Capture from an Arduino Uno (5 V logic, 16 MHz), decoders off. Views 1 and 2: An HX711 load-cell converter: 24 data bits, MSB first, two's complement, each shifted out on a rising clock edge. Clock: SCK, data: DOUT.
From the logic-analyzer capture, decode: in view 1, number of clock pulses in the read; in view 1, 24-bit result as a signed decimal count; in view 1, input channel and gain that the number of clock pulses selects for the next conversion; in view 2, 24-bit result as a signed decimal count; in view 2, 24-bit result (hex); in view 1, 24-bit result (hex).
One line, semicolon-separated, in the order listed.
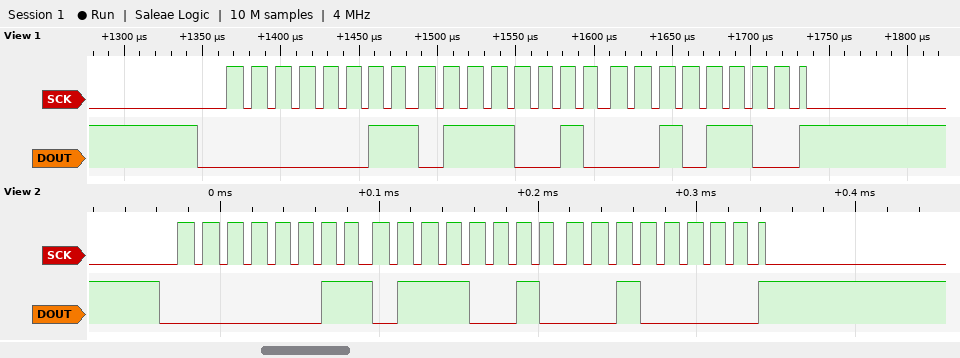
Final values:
25; 225836; channel A, gain 128; 225824; 0x037220; 0x03722C
